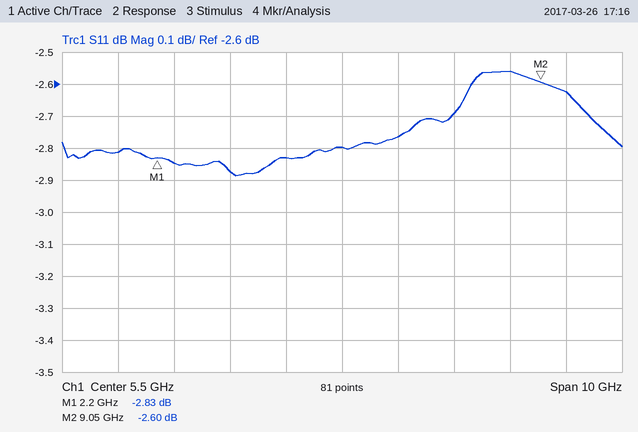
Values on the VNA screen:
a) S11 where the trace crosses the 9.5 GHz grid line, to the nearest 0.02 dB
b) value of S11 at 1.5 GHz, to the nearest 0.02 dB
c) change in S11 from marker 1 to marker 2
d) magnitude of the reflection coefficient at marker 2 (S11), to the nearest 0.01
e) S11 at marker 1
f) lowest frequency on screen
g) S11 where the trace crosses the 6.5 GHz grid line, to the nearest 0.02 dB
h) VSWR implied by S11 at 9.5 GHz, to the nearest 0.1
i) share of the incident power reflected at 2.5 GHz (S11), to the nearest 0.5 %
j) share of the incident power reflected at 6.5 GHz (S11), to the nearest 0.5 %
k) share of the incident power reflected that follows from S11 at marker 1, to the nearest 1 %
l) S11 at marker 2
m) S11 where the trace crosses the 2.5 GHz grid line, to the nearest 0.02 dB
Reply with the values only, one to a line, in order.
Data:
-2.62 dB
-2.82 dB
0.23 dB
0.74
-2.83 dB
500 MHz
-2.76 dB
6.7
52.0 %
53.0 %
52 %
-2.60 dB
-2.84 dB
